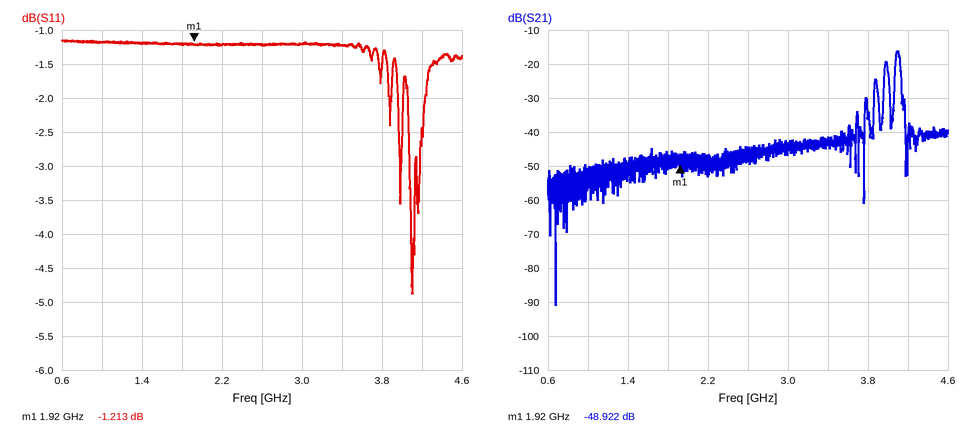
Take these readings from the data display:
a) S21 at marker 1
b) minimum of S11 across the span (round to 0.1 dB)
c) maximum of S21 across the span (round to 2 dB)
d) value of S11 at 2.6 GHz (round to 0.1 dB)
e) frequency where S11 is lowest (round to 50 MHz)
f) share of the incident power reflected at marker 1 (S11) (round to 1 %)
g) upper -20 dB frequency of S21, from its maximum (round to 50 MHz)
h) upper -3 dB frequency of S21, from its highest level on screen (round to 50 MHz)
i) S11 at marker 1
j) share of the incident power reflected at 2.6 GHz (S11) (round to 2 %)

-48.922 dB
-4.9 dB
-16 dB
-1.2 dB
4.10 GHz
76 %
4.15 GHz
4.10 GHz
-1.213 dB
76 %
